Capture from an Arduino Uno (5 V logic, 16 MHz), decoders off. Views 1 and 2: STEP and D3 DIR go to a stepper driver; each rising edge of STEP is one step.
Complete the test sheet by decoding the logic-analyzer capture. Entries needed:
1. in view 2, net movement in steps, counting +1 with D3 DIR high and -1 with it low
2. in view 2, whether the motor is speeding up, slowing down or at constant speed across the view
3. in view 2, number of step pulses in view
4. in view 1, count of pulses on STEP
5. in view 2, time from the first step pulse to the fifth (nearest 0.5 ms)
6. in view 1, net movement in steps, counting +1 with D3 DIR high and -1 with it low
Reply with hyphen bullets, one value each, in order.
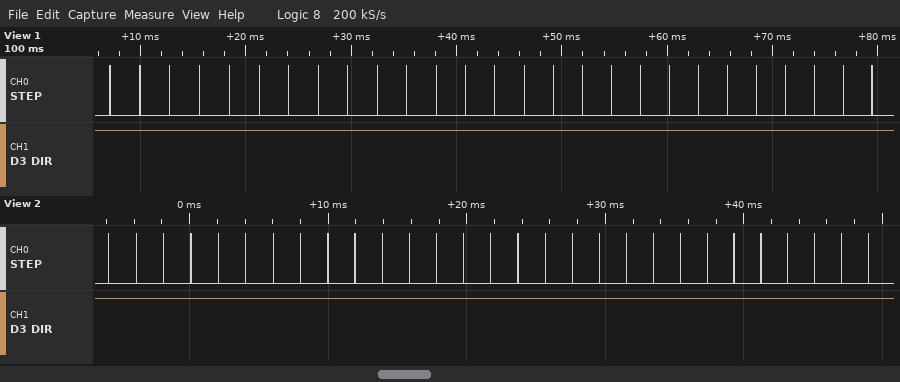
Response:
- +29
- constant speed
- 29
- 27
- 8.0 ms
- +27
